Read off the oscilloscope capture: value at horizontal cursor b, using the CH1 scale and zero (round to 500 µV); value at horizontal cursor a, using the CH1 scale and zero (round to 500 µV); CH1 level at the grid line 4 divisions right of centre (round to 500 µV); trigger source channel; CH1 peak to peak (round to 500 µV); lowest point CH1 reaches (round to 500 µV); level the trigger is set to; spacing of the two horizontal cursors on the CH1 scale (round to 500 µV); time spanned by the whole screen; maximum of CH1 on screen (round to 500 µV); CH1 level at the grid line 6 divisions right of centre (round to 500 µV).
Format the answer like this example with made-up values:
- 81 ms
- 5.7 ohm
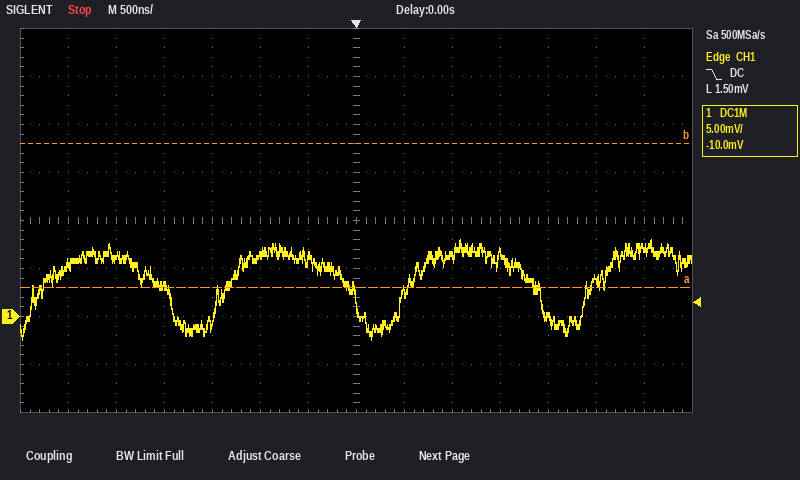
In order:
- 18.0 mV
- 3.0 mV
- 0.0 mV
- CH1
- 10.5 mV
- -2.5 mV
- 1.50 mV
- 15.0 mV
- 7 µs
- 8.0 mV
- 7.0 mV
